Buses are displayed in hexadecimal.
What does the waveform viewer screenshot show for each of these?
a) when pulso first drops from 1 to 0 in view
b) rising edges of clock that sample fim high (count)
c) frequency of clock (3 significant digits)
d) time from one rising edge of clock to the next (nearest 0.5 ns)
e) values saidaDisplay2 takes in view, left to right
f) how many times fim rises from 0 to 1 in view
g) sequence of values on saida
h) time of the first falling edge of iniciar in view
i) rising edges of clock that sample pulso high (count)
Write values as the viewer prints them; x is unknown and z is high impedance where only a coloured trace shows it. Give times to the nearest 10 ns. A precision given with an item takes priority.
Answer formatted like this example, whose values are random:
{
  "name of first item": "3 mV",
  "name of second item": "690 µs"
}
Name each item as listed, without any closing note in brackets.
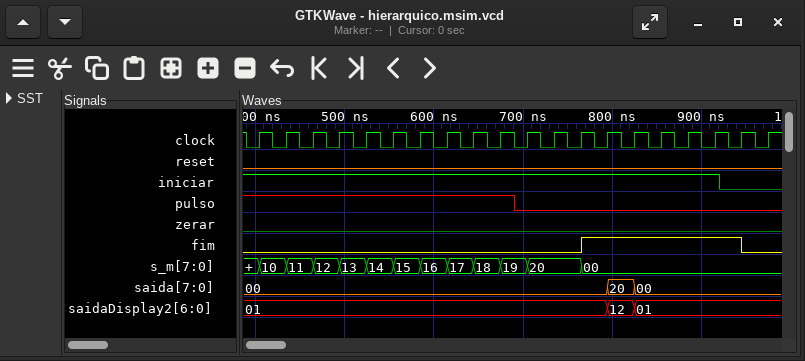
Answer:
{
  "when pulso first drops from 1 to 0 in view": "690 ns",
  "rising edges of clock that sample fim high": "6",
  "frequency of clock": "33.3 MHz",
  "time from one rising edge of clock to the next": "30 ns",
  "values saidaDisplay2 takes in view, left to right": "01, 12, 01",
  "how many times fim rises from 0 to 1 in view": "1",
  "sequence of values on saida": "00, 20, 00",
  "time of the first falling edge of iniciar in view": "920 ns",
  "rising edges of clock that sample pulso high": "10"
}
